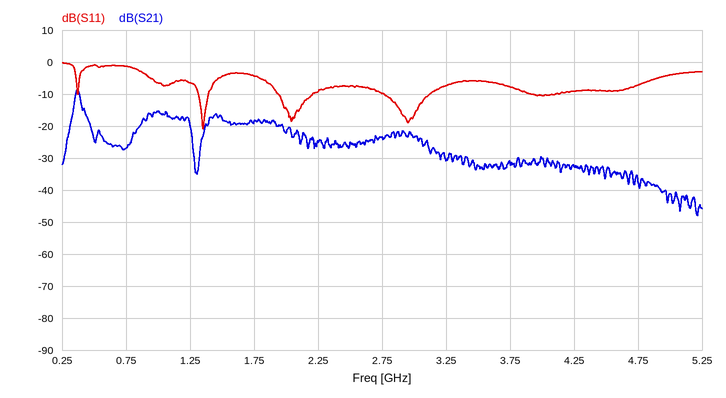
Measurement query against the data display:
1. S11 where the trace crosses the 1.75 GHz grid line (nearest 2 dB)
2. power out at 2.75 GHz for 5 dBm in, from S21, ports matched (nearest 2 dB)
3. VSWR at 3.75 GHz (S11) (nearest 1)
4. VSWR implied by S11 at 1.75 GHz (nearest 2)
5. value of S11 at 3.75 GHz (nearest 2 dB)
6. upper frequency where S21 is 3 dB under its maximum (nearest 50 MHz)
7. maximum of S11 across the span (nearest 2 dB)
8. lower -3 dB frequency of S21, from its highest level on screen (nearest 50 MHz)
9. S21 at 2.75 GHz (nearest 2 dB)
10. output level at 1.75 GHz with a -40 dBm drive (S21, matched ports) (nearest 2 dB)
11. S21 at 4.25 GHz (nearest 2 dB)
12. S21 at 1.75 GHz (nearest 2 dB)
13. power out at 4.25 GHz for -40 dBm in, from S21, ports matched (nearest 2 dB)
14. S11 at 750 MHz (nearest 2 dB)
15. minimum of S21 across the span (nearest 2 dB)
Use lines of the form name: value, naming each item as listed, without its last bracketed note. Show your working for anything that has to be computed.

S11 where the trace crosses the 1.75 GHz grid line: -4 dB
power out at 2.75 GHz for 5 dBm in, from S21, ports matched: 5 dBm + (-24 dB) = -18 dBm
VSWR at 3.75 GHz (S11): |Γ| = 10^(-8/20) = 0.3981; VSWR = (1 + 0.3981)/(1 − 0.3981) ≈ 2
VSWR implied by S11 at 1.75 GHz: |Γ| = 10^(-4/20) = 0.6310; VSWR = (1 + 0.6310)/(1 − 0.6310) ≈ 4
value of S11 at 3.75 GHz: -8 dB
upper frequency where S21 is 3 dB under its maximum: 400 MHz
maximum of S11 across the span: 0 dB
lower -3 dB frequency of S21, from its highest level on screen: 350 MHz
S21 at 2.75 GHz: -24 dB
output level at 1.75 GHz with a -40 dBm drive (S21, matched ports): -40 dBm + (-18 dB) = -58 dBm
S21 at 4.25 GHz: -32 dB
S21 at 1.75 GHz: -18 dB
power out at 4.25 GHz for -40 dBm in, from S21, ports matched: -40 dBm + (-32 dB) = -72 dBm
S11 at 750 MHz: -2 dB
minimum of S21 across the span: -48 dB
